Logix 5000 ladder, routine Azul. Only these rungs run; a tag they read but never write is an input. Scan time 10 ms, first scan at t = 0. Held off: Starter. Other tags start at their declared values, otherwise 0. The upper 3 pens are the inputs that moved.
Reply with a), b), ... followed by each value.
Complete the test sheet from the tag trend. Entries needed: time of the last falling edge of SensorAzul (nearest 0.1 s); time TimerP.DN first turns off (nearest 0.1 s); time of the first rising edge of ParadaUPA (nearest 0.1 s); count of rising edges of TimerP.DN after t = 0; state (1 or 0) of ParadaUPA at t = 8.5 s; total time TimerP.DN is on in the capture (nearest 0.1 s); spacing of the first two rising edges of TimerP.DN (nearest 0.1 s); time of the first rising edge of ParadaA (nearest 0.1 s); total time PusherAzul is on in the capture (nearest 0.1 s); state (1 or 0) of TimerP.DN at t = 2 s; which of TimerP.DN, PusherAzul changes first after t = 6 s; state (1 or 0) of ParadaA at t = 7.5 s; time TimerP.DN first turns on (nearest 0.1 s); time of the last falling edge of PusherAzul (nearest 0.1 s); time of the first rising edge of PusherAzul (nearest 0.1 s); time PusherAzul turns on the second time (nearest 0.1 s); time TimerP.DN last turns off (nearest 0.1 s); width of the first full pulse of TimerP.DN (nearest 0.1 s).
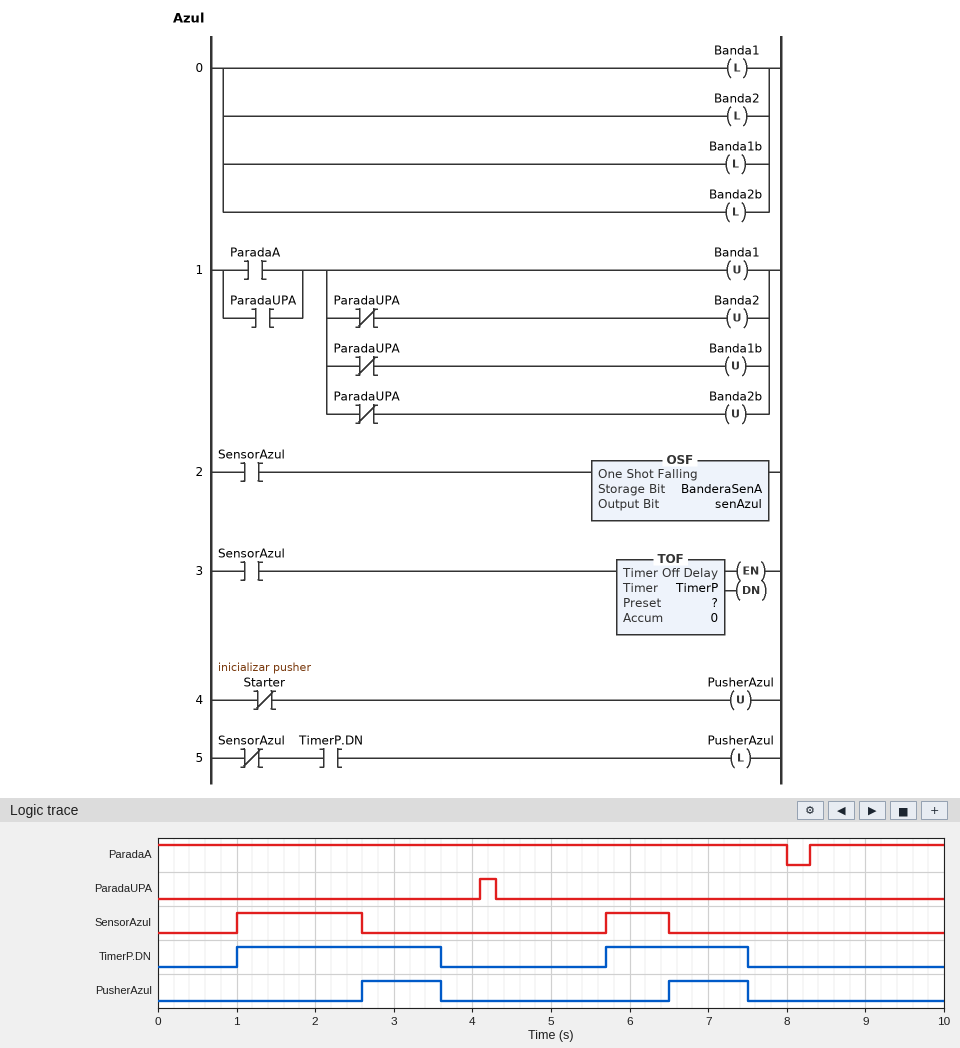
a) 6.5 s
b) 3.6 s
c) 4.1 s
d) 2
e) 0
f) 4.4 s
g) 4.7 s
h) 8.3 s
i) 2.0 s
j) 1
k) PusherAzul
l) 1
m) 1.0 s
n) 7.5 s
o) 2.6 s
p) 6.5 s
q) 7.5 s
r) 2.6 s
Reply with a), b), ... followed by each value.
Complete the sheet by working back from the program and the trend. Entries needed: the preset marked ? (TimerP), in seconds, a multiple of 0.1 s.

a) 1.0 s
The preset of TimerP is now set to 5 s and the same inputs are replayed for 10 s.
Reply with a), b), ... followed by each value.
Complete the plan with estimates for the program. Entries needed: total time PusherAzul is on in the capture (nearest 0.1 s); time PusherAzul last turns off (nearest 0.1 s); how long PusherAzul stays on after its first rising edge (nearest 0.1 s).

a) 6.6 s
b) 5.7 s
c) 3.1 s
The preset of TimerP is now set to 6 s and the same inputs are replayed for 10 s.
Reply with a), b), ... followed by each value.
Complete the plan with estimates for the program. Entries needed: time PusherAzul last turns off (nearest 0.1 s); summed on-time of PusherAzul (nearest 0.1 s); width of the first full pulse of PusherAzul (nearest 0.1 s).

a) 5.7 s
b) 6.6 s
c) 3.1 s
